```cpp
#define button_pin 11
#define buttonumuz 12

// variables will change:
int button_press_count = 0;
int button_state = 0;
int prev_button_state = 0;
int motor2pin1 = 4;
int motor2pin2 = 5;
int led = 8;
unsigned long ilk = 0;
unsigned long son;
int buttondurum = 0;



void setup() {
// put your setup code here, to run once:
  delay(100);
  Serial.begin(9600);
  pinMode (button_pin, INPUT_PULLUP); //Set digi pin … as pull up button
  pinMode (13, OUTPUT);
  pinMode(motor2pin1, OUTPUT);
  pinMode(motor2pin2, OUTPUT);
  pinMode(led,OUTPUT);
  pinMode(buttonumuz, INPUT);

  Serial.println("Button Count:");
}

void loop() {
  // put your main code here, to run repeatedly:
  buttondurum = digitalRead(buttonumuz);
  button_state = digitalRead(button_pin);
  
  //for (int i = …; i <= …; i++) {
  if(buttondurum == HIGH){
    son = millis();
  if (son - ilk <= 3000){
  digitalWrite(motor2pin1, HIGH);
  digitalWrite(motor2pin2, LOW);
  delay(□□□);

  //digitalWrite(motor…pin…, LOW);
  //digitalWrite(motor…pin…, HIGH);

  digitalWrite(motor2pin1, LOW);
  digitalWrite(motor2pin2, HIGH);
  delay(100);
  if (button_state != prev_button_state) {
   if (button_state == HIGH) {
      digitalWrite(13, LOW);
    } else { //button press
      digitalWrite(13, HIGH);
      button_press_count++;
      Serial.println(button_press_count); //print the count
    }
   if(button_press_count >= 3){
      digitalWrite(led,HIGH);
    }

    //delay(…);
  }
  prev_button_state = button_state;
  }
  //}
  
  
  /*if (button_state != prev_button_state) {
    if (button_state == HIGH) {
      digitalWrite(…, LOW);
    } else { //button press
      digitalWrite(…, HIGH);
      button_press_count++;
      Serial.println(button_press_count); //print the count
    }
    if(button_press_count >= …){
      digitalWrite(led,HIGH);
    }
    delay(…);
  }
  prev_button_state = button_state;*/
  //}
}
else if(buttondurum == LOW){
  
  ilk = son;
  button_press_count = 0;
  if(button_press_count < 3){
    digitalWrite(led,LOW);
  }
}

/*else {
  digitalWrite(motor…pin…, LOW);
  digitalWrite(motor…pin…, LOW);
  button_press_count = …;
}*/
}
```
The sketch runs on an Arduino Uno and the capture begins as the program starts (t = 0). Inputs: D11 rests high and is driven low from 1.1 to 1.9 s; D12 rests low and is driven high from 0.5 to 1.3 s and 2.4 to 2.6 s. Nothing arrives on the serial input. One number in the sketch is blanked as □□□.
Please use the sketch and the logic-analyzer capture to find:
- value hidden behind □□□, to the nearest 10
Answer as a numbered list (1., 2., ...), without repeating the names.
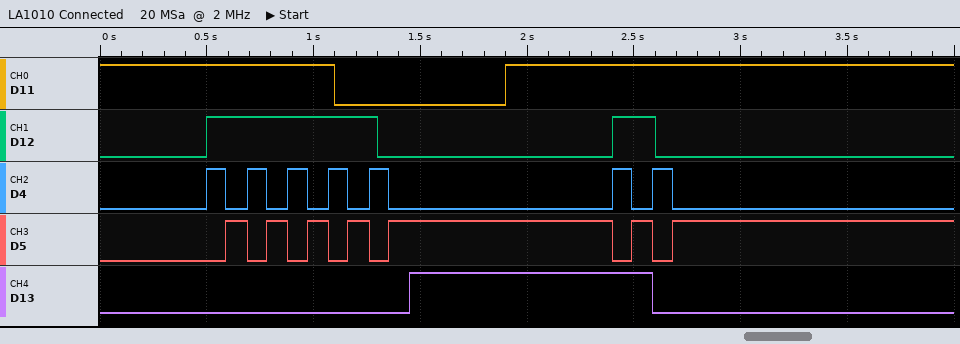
1. 90
